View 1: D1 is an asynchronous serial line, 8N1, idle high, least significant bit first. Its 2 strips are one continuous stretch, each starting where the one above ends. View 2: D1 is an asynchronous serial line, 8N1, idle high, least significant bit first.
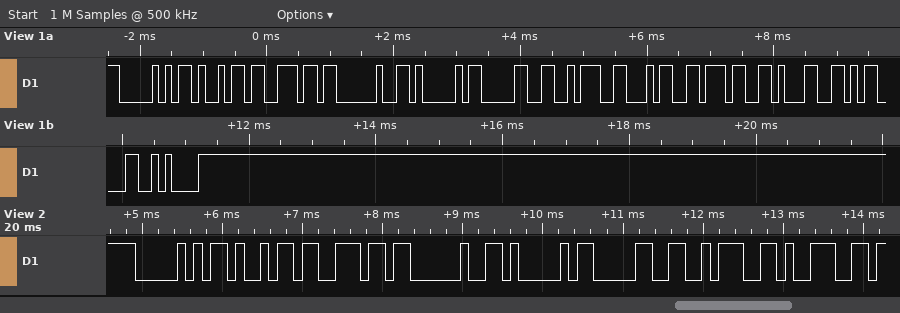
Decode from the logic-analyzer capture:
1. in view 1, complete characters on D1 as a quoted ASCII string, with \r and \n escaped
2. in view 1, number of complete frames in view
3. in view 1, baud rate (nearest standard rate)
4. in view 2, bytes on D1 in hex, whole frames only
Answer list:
"Pin A0:471\r\n"
12
9600 baud
0x50 0x69 0x6E 0x20 0x41 0x30 0x3A 0x39
